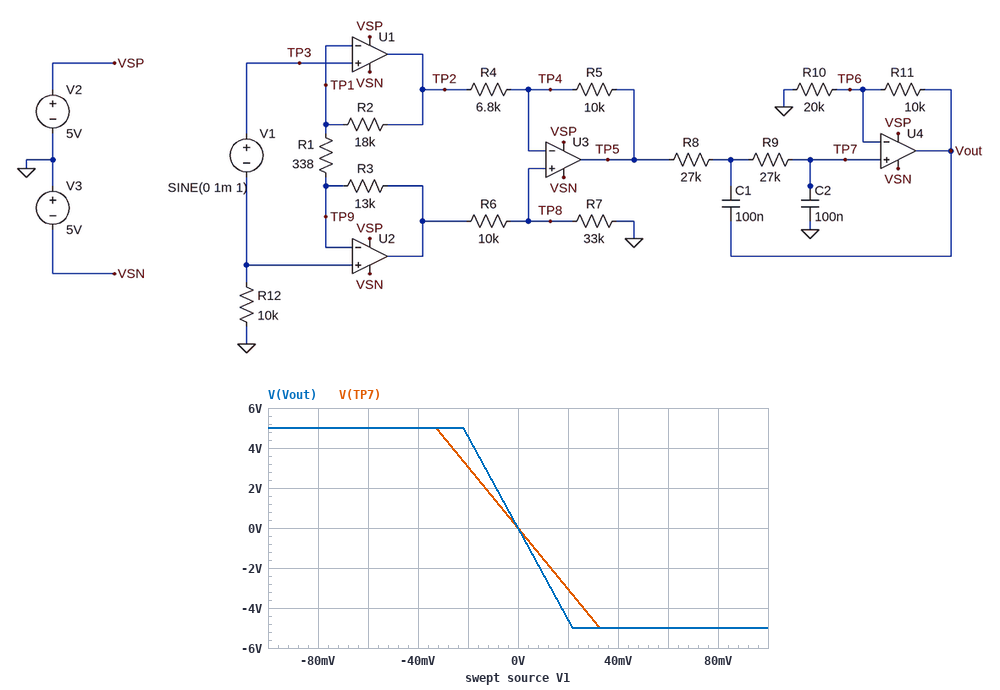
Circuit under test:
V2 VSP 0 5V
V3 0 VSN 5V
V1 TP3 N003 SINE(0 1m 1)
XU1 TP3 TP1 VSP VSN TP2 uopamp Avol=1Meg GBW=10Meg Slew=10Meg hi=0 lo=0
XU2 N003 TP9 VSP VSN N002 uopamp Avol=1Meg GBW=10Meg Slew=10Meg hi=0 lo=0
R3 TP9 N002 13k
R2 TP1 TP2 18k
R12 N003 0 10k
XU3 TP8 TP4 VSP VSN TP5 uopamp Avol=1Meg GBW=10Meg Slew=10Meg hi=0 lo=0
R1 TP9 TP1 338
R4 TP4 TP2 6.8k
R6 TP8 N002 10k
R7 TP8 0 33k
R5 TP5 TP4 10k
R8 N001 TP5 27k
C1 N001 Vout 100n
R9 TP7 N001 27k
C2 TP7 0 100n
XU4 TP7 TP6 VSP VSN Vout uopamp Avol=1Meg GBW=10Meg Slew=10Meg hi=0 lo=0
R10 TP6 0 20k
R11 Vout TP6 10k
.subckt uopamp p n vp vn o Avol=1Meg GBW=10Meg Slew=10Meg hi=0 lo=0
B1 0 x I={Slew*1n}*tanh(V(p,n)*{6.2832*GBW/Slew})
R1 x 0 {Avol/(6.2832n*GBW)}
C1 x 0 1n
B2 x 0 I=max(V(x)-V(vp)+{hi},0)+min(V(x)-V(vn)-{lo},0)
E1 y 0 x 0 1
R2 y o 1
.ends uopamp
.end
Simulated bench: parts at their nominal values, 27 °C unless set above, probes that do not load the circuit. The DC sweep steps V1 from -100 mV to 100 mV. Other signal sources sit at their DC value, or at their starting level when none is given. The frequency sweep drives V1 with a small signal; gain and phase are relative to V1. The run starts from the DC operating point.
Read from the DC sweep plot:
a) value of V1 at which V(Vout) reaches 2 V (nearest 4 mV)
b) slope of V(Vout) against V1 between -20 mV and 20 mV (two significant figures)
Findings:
-8 mV
-230 V/V
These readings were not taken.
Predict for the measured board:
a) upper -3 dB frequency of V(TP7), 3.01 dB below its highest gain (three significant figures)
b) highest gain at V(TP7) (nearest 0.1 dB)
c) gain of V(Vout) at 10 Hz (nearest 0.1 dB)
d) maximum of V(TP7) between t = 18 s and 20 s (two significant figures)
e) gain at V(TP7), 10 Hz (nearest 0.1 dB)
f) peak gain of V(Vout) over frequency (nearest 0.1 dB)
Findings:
55.4 Hz
43.7 dB
47.2 dB
150 mV
43.6 dB
47.2 dB
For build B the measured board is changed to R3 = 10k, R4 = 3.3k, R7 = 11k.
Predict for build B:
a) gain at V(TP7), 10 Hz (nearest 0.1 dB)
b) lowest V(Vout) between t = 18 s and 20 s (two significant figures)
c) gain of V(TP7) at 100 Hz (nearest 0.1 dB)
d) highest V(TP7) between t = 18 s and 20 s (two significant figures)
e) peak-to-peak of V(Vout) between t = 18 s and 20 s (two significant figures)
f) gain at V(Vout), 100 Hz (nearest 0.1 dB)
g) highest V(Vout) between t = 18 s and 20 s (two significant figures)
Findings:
47.1 dB
-340 mV
37.1 dB
230 mV
680 mV
40.6 dB
340 mV
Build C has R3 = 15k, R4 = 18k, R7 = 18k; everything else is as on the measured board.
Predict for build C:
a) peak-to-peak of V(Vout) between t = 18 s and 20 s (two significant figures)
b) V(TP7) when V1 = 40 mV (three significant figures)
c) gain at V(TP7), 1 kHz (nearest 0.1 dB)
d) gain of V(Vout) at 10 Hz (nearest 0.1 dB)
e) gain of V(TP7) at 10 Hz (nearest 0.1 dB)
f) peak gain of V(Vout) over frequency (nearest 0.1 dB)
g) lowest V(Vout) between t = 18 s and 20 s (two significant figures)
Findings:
220 mV
-2.98 V
-11.7 dB
40.9 dB
37.4 dB
41.0 dB
-110 mV
